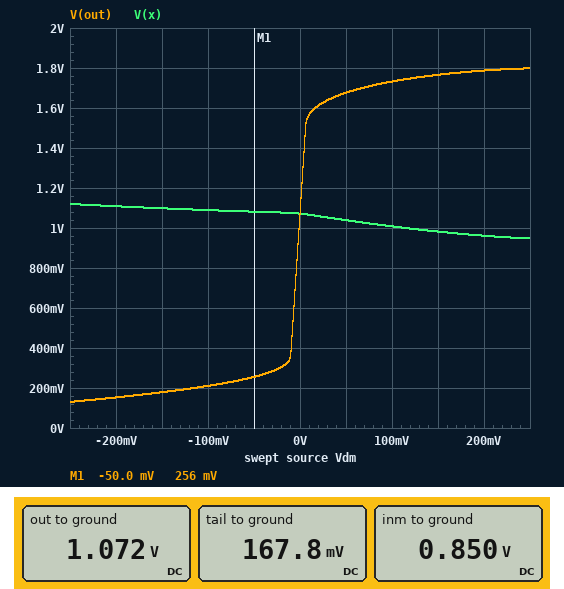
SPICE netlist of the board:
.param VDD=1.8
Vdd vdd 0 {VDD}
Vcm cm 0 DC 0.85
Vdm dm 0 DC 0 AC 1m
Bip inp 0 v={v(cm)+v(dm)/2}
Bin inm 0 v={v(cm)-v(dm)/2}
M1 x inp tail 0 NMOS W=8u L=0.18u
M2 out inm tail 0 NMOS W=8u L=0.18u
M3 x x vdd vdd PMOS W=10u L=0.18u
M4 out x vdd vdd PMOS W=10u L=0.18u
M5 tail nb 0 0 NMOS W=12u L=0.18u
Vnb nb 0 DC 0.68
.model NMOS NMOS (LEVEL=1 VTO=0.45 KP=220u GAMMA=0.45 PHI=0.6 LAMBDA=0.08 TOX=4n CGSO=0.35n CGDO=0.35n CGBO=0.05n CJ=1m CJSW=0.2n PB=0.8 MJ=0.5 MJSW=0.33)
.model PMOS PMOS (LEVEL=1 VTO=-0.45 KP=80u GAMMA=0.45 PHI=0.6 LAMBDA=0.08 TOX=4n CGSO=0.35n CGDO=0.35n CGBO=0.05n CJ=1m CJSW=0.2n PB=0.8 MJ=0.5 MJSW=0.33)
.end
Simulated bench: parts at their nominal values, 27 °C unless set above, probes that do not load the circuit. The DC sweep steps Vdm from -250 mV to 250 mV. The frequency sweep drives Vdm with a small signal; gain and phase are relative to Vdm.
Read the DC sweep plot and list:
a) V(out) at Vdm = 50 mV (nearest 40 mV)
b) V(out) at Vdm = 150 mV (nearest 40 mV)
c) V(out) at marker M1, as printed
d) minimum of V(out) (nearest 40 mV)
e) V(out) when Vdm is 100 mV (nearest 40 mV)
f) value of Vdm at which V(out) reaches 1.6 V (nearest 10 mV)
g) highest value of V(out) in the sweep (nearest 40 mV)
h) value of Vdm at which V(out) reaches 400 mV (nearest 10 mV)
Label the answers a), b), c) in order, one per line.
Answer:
a) 1.68 V
b) 1.76 V
c) 256 mV
d) 120 mV
e) 1.72 V
f) 20 mV
g) 1.80 V
h) -10 mV
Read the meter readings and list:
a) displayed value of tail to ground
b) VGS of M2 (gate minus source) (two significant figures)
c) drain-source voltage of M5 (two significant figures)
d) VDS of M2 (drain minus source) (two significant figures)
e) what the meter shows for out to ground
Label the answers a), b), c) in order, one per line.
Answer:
a) 167.8 mV
b) 680 mV
c) 170 mV
d) 900 mV
e) 1.072 V
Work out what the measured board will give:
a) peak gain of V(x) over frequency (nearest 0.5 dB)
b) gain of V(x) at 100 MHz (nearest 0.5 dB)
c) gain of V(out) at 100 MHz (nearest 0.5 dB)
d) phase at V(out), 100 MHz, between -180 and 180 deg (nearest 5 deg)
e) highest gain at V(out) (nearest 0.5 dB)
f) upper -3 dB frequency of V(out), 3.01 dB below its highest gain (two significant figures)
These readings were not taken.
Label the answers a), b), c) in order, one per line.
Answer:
a) -7.5 dB
b) -7.5 dB
c) 37.0 dB
d) -15 deg
e) 37.0 dB
f) 440 MHz
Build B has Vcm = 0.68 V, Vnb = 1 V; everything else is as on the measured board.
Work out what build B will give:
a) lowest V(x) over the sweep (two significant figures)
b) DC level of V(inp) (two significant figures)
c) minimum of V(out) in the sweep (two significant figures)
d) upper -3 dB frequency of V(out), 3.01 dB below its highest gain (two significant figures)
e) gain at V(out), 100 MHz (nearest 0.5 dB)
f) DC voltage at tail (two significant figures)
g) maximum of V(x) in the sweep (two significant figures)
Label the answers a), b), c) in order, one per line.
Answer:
a) 930 mV
b) 680 mV
c) 26 mV
d) 390 MHz
e) 37.5 dB
f) 42 mV
g) 1.2 V
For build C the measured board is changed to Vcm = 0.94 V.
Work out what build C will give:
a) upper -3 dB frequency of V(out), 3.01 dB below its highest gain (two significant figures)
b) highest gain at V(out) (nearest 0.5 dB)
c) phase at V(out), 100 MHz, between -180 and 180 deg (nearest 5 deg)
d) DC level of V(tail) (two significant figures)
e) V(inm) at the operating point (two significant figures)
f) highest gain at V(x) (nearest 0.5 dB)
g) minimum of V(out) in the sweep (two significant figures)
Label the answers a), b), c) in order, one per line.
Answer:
a) 480 MHz
b) 36.5 dB
c) -10 deg
d) 230 mV
e) 940 mV
f) -8.5 dB
g) 190 mV
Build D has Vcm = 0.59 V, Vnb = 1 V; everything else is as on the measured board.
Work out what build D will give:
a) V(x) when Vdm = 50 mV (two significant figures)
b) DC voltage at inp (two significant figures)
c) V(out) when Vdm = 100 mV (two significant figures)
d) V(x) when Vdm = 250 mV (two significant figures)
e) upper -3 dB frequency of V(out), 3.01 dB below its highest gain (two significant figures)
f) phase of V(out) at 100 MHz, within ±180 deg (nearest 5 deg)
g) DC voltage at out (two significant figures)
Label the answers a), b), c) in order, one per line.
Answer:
a) 1.1 V
b) 590 mV
c) 1.8 V
d) 1.0 V
e) 170 MHz
f) -30 deg
g) 1.2 V
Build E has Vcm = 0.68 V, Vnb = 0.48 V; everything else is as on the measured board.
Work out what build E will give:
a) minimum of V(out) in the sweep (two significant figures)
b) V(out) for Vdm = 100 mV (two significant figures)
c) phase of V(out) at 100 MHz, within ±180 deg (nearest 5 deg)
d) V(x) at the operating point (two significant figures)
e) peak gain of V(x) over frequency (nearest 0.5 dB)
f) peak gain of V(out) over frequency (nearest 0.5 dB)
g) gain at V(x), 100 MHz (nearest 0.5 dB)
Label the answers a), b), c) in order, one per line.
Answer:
a) 64 mV
b) 1.8 V
c) -85 deg
d) 1.3 V
e) -8.0 dB
f) 54.5 dB
g) -13.0 dB
